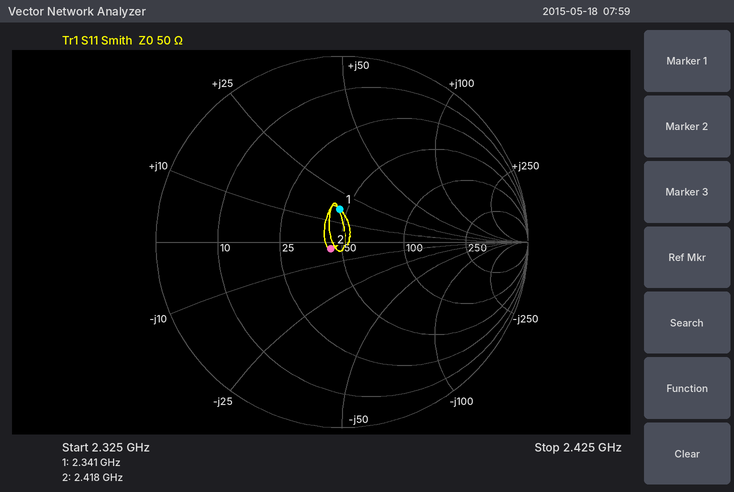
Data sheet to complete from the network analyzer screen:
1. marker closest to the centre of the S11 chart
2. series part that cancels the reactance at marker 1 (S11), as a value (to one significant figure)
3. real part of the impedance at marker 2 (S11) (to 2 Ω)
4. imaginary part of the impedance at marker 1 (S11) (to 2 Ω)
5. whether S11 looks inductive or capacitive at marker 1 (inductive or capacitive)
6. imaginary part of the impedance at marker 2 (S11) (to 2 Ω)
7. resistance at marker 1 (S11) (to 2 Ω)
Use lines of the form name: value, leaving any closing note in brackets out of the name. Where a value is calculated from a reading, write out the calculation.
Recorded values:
marker closest to the centre of the S11 chart: marker 2
series part that cancels the reactance at marker 1 (S11), as a value: C = 1/(2π × 2.341 GHz × 16 Ω) ≈ 4 pF
real part of the impedance at marker 2 (S11): 44 Ω
imaginary part of the impedance at marker 1 (S11): +16 Ω
whether S11 looks inductive or capacitive at marker 1: inductive
imaginary part of the impedance at marker 2 (S11): -4 Ω
resistance at marker 1 (S11): 46 Ω
